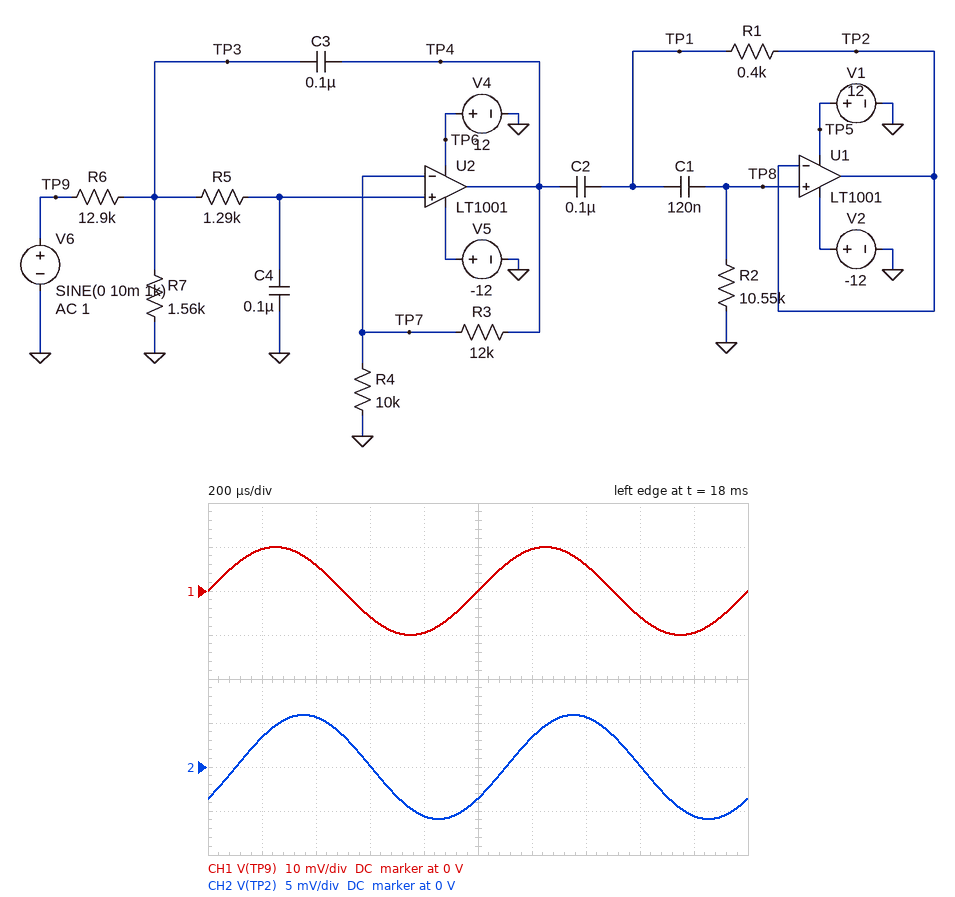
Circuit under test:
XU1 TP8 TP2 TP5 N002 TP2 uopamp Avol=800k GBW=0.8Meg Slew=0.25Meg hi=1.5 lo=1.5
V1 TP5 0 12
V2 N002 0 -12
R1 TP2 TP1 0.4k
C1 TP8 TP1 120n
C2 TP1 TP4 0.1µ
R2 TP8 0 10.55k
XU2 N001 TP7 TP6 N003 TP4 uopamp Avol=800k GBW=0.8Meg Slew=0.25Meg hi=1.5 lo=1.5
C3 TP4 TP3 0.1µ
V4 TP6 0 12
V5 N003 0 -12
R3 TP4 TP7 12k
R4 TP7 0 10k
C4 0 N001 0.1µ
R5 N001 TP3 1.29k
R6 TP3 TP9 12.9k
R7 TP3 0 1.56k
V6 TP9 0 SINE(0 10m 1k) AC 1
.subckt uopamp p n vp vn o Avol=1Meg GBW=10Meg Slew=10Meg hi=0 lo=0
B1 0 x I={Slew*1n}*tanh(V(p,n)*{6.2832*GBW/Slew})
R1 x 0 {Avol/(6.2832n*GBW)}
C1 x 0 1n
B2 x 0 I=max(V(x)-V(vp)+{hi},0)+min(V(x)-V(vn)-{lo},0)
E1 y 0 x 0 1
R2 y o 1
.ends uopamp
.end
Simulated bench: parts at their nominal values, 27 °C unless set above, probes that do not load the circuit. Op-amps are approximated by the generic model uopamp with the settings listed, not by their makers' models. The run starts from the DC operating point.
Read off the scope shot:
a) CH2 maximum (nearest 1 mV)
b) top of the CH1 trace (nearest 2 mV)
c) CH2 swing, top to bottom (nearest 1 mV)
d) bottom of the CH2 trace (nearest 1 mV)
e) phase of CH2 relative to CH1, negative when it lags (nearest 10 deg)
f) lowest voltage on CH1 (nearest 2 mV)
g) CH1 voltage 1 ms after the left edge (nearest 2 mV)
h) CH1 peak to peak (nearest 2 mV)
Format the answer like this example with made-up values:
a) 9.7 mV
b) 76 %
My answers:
a) 6 mV
b) 10 mV
c) 12 mV
d) -6 mV
e) -40 deg
f) -10 mV
g) 0 V
h) 20 mV
